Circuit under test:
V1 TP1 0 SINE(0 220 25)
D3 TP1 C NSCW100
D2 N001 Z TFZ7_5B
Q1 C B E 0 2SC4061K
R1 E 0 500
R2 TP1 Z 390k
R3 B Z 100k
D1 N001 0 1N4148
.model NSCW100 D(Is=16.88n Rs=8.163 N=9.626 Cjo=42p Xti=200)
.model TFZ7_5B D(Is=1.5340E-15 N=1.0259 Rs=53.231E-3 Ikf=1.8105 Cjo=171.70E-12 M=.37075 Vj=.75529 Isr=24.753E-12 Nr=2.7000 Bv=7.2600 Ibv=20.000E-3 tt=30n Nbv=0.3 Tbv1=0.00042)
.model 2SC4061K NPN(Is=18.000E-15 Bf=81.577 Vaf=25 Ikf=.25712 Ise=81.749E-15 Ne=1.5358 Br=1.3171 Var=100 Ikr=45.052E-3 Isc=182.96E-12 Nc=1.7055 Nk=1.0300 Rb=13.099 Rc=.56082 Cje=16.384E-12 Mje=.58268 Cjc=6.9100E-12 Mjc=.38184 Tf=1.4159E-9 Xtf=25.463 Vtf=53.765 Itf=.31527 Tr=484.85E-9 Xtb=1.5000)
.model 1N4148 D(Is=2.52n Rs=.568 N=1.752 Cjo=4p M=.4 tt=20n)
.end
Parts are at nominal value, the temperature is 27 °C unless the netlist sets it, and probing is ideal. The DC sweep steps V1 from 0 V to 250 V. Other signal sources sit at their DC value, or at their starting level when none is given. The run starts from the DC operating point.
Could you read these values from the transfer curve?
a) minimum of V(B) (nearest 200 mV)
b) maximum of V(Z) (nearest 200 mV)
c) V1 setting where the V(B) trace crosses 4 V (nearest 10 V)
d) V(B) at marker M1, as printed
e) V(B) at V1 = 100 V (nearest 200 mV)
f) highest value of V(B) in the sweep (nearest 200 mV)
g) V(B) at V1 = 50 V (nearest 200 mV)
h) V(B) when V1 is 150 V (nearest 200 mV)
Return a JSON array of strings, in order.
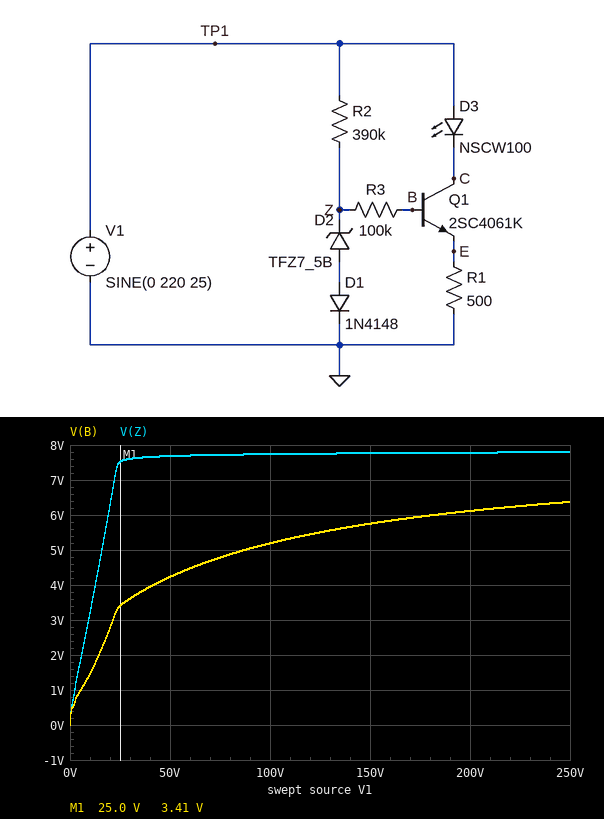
["0 V", "7.8 V", "40 V", "3.41 V", "5.2 V", "6.4 V", "4.2 V", "5.8 V"]
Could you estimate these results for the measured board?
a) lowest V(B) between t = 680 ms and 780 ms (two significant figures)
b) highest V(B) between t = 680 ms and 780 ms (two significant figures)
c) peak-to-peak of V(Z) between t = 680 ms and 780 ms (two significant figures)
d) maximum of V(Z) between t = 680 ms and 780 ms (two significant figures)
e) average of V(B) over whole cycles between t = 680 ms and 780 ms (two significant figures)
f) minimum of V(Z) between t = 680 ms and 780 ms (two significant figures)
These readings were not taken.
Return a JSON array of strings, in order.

["-220 V", "6.2 V", "230 V", "7.8 V", "-67 V", "-220 V"]
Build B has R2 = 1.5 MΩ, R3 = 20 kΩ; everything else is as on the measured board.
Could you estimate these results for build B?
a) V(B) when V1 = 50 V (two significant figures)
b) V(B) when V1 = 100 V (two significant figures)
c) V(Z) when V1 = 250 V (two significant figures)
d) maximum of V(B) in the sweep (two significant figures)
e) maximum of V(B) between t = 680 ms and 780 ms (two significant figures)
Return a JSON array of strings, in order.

["3.8 V", "6.9 V", "7.7 V", "7.4 V", "7.3 V"]
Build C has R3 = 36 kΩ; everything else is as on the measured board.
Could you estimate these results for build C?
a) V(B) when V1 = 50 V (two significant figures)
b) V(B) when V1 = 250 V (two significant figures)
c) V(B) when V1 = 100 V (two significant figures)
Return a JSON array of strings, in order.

["5.8 V", "7.2 V", "6.5 V"]
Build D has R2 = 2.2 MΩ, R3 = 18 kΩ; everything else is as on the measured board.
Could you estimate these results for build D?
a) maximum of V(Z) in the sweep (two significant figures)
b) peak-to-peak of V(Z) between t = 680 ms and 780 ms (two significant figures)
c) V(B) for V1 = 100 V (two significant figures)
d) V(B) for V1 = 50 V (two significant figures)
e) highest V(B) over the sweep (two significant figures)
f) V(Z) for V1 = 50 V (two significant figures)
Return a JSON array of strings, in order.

["7.7 V", "230 V", "6.9 V", "2.9 V", "7.4 V", "3.3 V"]
